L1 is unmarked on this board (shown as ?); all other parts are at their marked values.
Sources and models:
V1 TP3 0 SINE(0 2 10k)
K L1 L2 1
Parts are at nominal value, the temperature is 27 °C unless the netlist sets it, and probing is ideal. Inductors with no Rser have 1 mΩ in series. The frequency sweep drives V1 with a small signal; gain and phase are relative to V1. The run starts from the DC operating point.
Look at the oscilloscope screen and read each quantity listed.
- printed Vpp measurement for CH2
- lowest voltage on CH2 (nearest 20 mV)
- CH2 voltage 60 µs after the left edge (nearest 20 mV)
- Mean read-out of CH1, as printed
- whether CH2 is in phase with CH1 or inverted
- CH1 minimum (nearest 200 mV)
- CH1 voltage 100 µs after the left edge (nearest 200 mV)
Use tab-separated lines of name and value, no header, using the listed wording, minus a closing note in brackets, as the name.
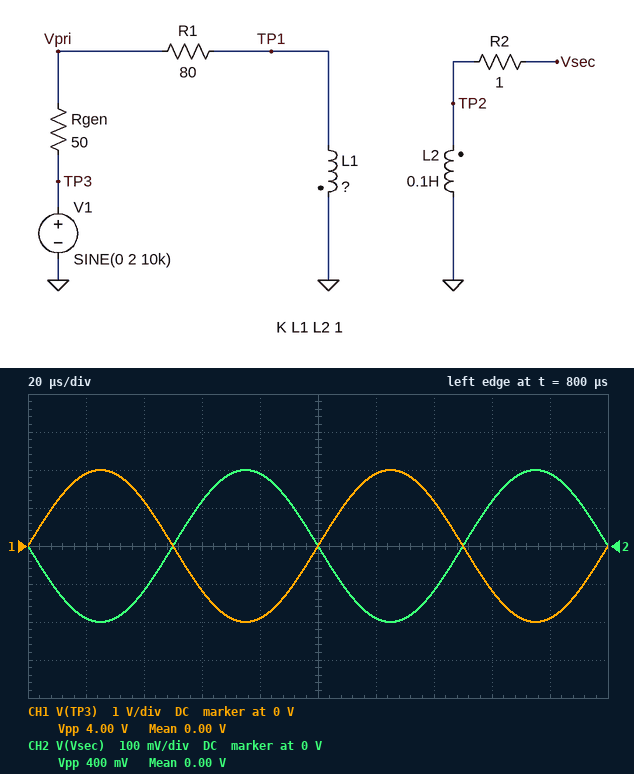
printed Vpp measurement for CH2	400 mV
lowest voltage on CH2	-200 mV
CH2 voltage 60 µs after the left edge	120 mV
Mean read-out of CH1, as printed	0.00 V
whether CH2 is in phase with CH1 or inverted	inverted
CH1 minimum	-2.0 V
CH1 voltage 100 µs after the left edge	0 V
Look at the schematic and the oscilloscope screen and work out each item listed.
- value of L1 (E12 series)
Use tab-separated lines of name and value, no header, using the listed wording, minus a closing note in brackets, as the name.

value of L1	10 H
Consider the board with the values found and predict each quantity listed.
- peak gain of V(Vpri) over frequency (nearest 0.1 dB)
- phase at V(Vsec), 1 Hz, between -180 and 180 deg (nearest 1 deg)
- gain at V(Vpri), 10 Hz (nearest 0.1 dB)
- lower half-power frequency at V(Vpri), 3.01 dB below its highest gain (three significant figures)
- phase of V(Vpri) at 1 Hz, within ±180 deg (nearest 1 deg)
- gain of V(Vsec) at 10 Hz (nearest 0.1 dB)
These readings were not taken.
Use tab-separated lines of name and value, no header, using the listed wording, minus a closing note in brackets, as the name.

peak gain of V(Vpri) over frequency	0 dB
phase at V(Vsec), 1 Hz, between -180 and 180 deg	-116 deg
gain at V(Vpri), 10 Hz	-0.1 dB
lower half-power frequency at V(Vpri), 3.01 dB below its highest gain	1.02 Hz
phase of V(Vpri) at 1 Hz, within ±180 deg	12 deg
gain of V(Vsec) at 10 Hz	-20.2 dB
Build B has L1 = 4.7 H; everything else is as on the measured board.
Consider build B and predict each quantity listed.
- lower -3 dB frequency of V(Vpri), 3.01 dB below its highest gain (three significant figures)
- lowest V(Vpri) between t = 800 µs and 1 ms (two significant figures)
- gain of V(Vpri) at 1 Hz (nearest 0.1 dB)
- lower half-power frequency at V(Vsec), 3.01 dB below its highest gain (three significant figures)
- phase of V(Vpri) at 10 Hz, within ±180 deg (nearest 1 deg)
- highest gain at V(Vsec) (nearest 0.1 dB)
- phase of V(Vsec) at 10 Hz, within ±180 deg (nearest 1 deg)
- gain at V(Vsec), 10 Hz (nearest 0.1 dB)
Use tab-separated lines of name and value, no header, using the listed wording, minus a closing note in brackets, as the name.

lower -3 dB frequency of V(Vpri), 3.01 dB below its highest gain	2.17 Hz
lowest V(Vpri) between t = 800 µs and 1 ms	-2.0 V
gain of V(Vpri) at 1 Hz	-3.9 dB
lower half-power frequency at V(Vsec), 3.01 dB below its highest gain	4.40 Hz
phase of V(Vpri) at 10 Hz, within ±180 deg	9 deg
highest gain at V(Vsec)	-16.7 dB
phase of V(Vsec) at 10 Hz, within ±180 deg	-156 deg
gain at V(Vsec), 10 Hz	-17.5 dB
